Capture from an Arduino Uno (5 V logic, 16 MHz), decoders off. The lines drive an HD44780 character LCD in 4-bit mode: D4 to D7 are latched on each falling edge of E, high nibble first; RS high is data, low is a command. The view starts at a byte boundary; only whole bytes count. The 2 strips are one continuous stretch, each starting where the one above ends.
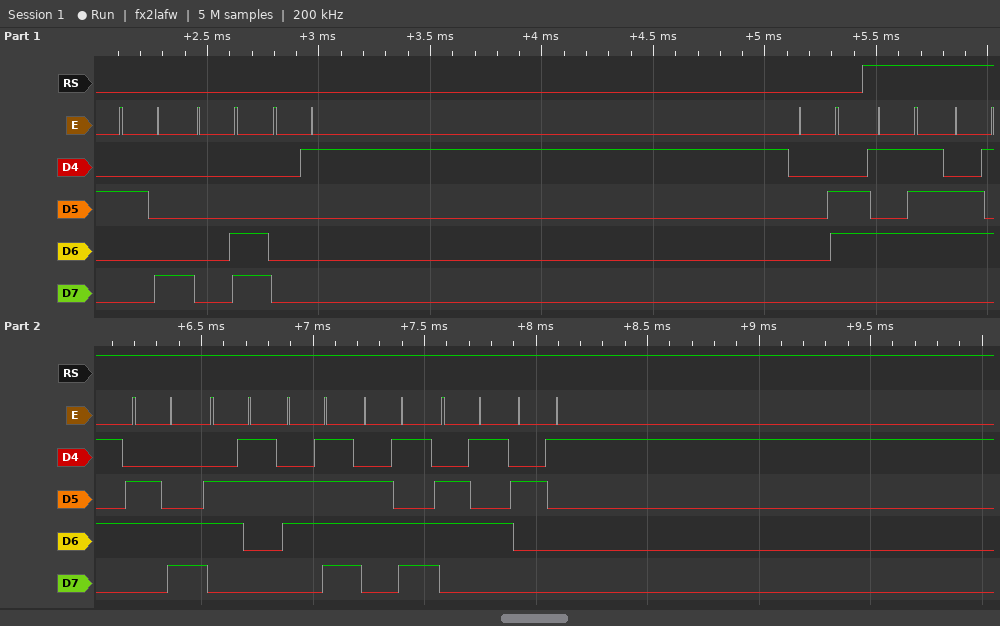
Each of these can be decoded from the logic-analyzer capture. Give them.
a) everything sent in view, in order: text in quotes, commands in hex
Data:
0x28 0x0C 0x01 0x06 "Welcome!"
